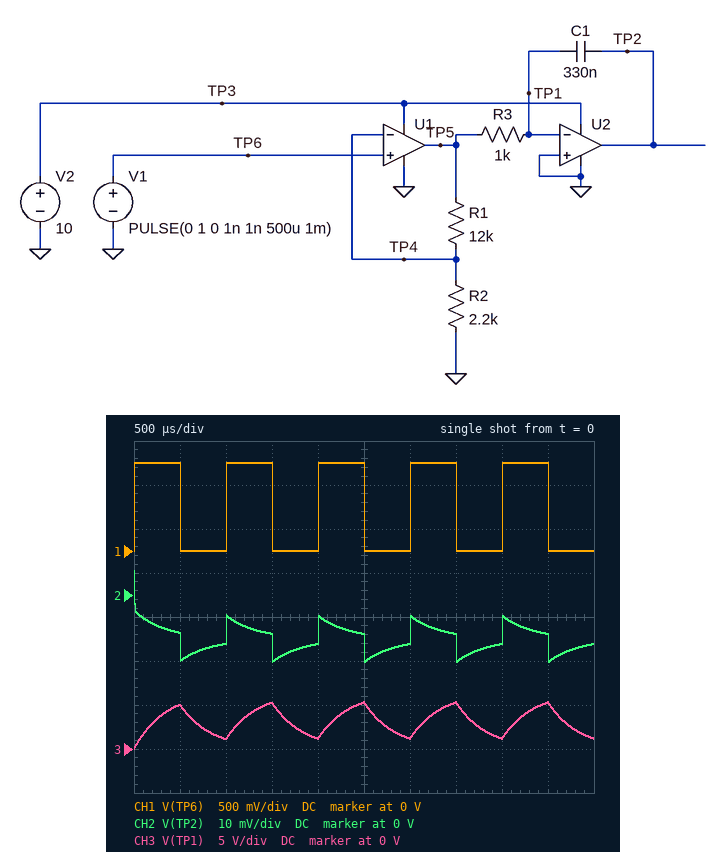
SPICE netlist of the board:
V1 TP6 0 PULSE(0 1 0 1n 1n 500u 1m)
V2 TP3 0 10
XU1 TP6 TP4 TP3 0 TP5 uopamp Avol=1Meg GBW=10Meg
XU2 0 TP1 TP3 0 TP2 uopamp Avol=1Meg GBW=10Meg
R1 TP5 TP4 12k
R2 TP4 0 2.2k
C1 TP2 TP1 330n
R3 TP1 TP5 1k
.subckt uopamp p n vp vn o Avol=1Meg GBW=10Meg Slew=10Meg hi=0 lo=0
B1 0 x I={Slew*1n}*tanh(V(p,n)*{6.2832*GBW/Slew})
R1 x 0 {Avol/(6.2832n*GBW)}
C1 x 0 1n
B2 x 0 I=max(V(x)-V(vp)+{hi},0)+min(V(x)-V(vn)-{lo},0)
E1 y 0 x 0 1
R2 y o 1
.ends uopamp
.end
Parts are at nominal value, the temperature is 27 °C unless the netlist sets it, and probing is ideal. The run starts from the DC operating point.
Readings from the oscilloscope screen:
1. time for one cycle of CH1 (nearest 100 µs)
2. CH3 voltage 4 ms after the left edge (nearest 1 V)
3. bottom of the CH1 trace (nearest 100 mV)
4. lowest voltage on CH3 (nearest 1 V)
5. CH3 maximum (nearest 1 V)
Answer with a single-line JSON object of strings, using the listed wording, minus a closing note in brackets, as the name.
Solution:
{"time for one cycle of CH1": "1.0 ms", "CH3 voltage 4 ms after the left edge": "1 V", "bottom of the CH1 trace": "0 V", "lowest voltage on CH3": "0 V", "CH3 maximum": "5 V"}
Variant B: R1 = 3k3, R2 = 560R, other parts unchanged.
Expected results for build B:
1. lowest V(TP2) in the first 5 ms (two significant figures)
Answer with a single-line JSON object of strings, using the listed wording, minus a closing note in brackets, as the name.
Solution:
{"lowest V(TP2) in the first 5 ms": "-16 mV"}
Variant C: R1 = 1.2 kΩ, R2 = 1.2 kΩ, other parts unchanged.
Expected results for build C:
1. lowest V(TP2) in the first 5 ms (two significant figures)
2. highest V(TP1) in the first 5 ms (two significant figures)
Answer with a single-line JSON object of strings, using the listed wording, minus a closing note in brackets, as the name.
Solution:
{"lowest V(TP2) in the first 5 ms": "-12 mV", "highest V(TP1) in the first 5 ms": "1.6 V"}
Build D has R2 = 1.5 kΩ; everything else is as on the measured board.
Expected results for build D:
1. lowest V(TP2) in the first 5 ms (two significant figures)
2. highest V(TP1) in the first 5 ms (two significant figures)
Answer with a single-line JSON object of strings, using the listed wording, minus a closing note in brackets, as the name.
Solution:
{"lowest V(TP2) in the first 5 ms": "-17 mV", "highest V(TP1) in the first 5 ms": "7.4 V"}
